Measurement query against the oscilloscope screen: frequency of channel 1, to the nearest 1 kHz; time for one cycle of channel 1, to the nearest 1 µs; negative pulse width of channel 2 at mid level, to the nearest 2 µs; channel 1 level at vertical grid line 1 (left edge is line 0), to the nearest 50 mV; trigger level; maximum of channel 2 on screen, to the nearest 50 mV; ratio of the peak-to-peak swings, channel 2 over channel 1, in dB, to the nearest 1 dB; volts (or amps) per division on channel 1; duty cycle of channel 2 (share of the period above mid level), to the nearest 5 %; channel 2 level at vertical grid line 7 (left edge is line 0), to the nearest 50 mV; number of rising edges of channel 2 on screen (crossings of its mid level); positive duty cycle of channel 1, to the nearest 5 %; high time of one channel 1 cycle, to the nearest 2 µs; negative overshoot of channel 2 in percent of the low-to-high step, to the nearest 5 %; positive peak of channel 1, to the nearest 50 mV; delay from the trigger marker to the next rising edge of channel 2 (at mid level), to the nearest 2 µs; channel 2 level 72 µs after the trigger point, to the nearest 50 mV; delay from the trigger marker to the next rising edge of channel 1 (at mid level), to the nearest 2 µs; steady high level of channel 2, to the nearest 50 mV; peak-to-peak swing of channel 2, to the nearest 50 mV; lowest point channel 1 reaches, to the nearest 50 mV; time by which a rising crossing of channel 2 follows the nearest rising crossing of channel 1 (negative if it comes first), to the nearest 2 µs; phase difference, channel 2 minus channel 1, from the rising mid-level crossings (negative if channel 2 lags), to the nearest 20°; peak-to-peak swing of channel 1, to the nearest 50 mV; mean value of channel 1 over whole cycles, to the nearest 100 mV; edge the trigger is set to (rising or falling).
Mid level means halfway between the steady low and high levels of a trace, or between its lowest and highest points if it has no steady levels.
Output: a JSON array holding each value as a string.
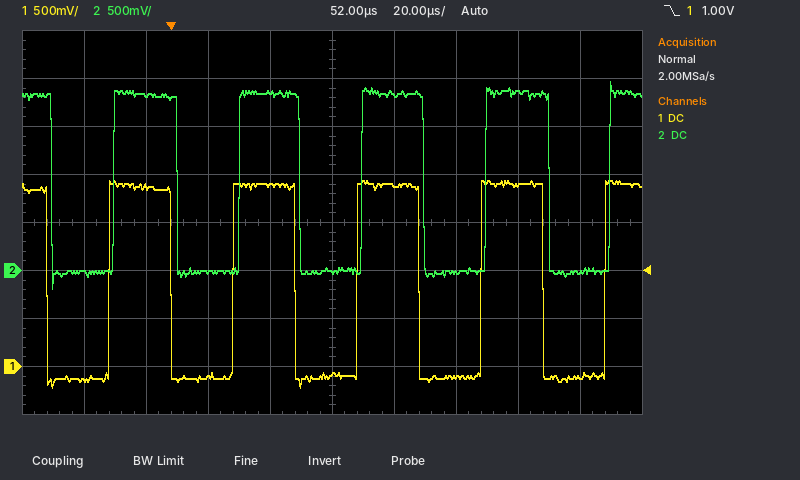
["25 kHz", "40 µs", "20 µs", "-150 mV", "1.00 V", "1.95 V", "0 dB", "500 mV", "50 %", "0 mV", "5", "50 %", "20 µs", "10 %", "1.95 V", "22 µs", "1.85 V", "20 µs", "1.85 V", "2.15 V", "-200 mV", "+2 µs", "-20°", "2.15 V", "900 mV", "falling"]
